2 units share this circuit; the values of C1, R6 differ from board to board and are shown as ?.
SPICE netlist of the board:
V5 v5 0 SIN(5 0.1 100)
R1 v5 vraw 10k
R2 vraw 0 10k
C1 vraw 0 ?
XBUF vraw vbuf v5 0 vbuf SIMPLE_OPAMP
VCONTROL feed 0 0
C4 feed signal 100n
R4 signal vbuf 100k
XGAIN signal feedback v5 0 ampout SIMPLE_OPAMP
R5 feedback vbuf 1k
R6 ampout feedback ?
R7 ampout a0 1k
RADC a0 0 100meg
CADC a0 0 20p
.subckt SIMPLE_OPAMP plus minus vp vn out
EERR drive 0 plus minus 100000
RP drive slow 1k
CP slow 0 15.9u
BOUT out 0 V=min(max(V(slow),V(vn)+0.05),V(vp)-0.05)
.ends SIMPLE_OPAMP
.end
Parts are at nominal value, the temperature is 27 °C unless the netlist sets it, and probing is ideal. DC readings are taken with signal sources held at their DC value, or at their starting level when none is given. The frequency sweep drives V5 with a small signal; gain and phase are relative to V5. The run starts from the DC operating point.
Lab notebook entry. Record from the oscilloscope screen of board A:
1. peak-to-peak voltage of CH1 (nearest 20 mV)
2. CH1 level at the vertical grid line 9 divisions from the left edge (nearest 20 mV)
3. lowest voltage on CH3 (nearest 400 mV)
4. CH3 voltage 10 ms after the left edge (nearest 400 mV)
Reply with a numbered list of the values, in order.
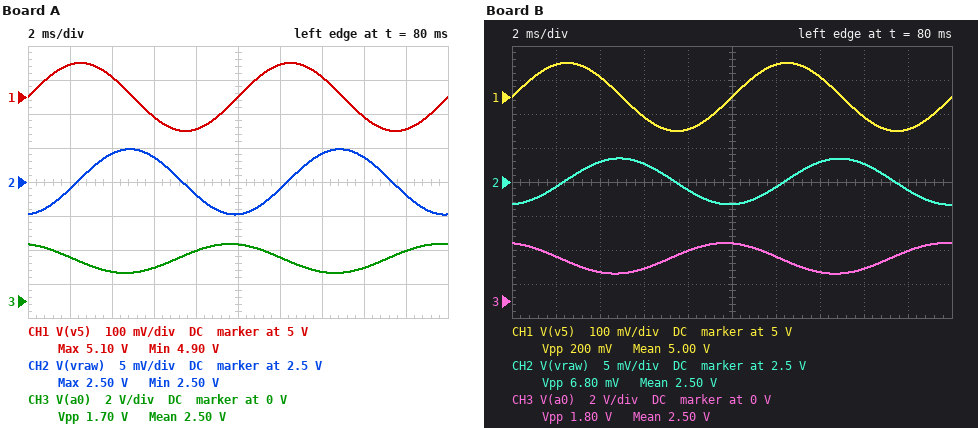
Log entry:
1. 200 mV
2. 4.90 V
3. 1.6 V
4. 3.2 V
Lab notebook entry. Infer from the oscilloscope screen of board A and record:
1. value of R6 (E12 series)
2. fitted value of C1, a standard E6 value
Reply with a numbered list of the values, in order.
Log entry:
1. 180 kΩ
2. 3.3 µF
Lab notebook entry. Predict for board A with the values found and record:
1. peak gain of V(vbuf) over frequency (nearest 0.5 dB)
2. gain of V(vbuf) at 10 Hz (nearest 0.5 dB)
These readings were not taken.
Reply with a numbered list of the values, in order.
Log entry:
1. -6.0 dB
2. -9.0 dB
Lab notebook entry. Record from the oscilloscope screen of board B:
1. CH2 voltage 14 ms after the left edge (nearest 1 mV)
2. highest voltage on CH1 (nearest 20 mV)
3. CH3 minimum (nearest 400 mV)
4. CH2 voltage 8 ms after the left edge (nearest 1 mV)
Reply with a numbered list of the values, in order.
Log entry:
1. 2.503 V
2. 5.10 V
3. 1.6 V
4. 2.499 V
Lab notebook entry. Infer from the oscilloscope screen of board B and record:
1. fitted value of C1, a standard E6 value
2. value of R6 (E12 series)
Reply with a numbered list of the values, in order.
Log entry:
1. 4.7 µF
2. 270 kΩ
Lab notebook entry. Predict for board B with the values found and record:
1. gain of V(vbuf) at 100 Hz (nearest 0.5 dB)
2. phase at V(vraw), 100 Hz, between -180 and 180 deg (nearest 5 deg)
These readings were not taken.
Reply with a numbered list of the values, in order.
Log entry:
1. -29.5 dB
2. -85 deg
